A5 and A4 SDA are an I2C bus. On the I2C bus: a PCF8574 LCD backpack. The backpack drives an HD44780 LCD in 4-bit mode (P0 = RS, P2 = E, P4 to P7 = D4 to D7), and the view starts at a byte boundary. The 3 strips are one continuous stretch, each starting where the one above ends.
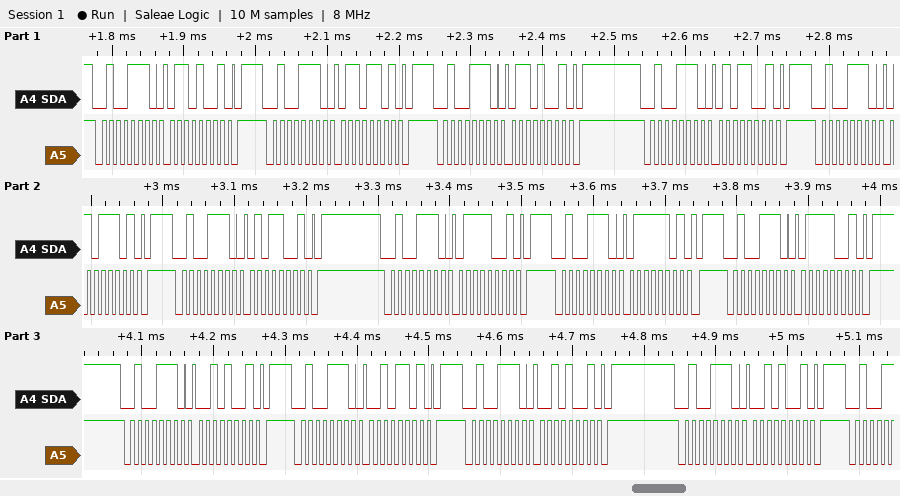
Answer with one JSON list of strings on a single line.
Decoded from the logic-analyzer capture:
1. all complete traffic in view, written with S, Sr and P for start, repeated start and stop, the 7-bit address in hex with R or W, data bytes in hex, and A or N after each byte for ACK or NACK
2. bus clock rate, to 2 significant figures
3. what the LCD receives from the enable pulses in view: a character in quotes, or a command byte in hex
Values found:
["S 27W A 69 A P S 27W A 6D A P S 27W A 69 A P S 27W A 59 A P S 27W A 5D A P S 27W A 59 A P S 27W A 79 A P S 27W A 7D A P S 27W A 79 A P S 27W A 29 A P S 27W A 2D A P S 27W A 29 A P S 27W A 29 A P", "100 kHz", "'e' 'r'"]
